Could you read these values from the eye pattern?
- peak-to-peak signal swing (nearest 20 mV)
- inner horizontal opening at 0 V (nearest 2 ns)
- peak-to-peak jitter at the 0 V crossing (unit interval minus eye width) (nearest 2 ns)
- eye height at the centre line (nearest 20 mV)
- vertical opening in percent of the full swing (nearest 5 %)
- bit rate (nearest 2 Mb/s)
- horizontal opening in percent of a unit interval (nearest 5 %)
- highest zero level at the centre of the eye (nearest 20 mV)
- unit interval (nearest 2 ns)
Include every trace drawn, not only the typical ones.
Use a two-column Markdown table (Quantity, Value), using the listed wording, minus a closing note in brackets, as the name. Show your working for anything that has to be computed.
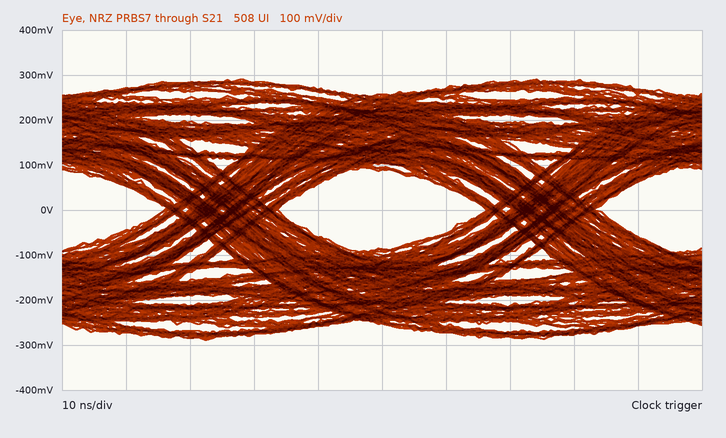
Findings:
| Quantity | Value |
|---|---|
| peak-to-peak signal swing | 580 mV |
| inner horizontal opening at 0 V | 32 ns |
| peak-to-peak jitter at the 0 V crossing (unit interval minus eye width) | 18 ns |
| eye height at the centre line | 180 mV |
| vertical opening in percent of the full swing | 180 mV / 580 mV ≈ 31.0 %, so 30 % to the nearest 5 % |
| bit rate | 20 Mb/s |
| horizontal opening in percent of a unit interval | 32 ns / 50 ns ≈ 64.0 %, so 65 % to the nearest 5 % |
| highest zero level at the centre of the eye | -80 mV |
| unit interval | 50 ns |
